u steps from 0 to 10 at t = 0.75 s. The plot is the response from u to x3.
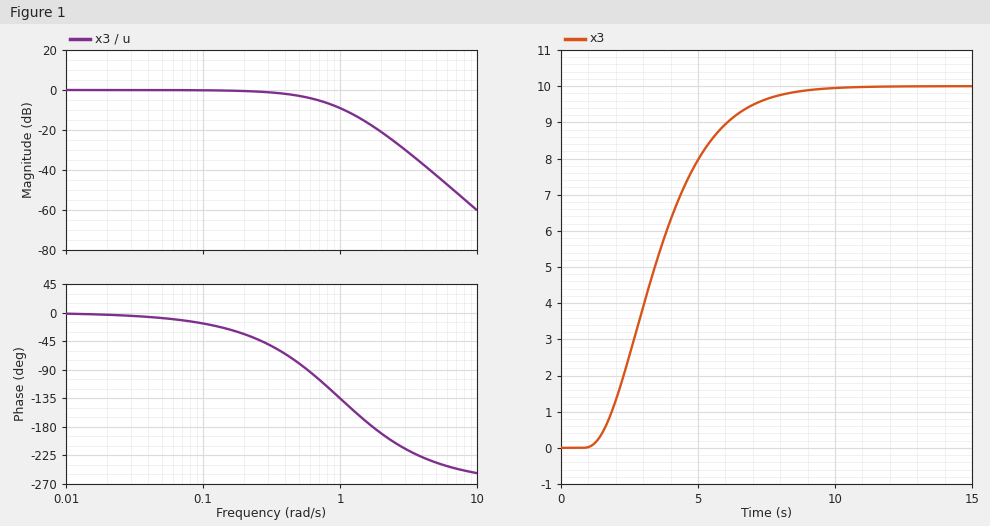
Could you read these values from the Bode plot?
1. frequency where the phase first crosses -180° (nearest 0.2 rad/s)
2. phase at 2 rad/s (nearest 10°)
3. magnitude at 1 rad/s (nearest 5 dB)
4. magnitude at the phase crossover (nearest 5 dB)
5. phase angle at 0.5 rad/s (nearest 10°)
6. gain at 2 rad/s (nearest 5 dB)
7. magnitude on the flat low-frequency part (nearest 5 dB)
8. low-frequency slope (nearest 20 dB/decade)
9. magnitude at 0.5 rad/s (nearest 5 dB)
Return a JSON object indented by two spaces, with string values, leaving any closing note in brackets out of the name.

{
  "frequency where the phase first crosses -180°": "1.8 rad/s",
  "phase at 2 rad/s": "-190°",
  "magnitude at 1 rad/s": "-10 dB",
  "magnitude at the phase crossover": "-20 dB",
  "phase angle at 0.5 rad/s": "-80°",
  "gain at 2 rad/s": "-20 dB",
  "magnitude on the flat low-frequency part": "0 dB",
  "low-frequency slope": "0 dB/decade",
  "magnitude at 0.5 rad/s": "-5 dB"
}
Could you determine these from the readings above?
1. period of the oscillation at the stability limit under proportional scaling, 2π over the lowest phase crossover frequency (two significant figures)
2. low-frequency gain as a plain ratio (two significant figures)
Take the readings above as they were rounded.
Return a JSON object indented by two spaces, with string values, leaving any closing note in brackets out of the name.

{
  "period of the oscillation at the stability limit under proportional scaling, 2π over the lowest phase crossover frequency": "3.5 s",
  "low-frequency gain as a plain ratio": "1.0"
}
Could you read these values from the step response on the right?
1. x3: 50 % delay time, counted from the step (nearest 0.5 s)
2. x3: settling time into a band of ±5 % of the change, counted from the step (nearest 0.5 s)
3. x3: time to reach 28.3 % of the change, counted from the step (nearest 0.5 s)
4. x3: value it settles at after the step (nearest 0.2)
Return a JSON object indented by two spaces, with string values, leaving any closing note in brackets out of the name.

{
  "x3: 50 % delay time, counted from the step": "2.5 s",
  "x3: settling time into a band of ±5 % of the change, counted from the step": "6.5 s",
  "x3: time to reach 28.3 % of the change, counted from the step": "2.0 s",
  "x3: value it settles at after the step": "10.0"
}
